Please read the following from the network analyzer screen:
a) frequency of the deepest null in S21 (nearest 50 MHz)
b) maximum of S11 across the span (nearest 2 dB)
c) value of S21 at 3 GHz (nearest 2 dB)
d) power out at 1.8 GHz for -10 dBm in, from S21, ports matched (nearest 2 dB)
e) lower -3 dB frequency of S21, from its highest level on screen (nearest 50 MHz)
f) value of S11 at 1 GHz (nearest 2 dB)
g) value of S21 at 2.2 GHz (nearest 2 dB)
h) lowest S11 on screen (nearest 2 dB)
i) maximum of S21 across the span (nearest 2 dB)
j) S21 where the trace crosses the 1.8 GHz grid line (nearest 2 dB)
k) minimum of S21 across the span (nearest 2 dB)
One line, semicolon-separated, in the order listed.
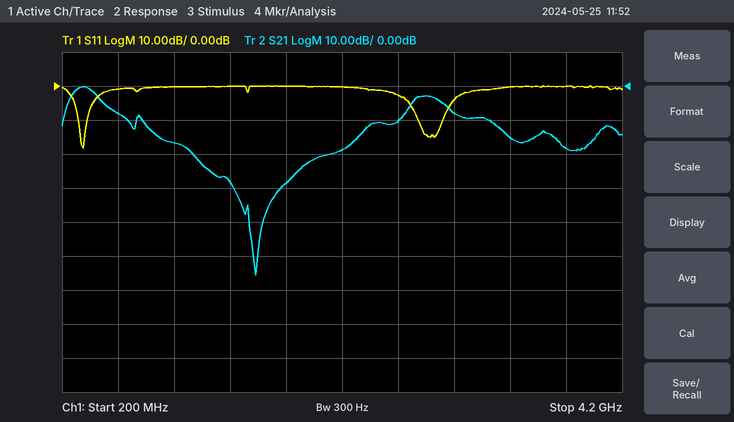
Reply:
1.60 GHz; 0 dB; -8 dB; -38 dBm; 250 MHz; 0 dB; -18 dB; -18 dB; 0 dB; -28 dB; -56 dB
